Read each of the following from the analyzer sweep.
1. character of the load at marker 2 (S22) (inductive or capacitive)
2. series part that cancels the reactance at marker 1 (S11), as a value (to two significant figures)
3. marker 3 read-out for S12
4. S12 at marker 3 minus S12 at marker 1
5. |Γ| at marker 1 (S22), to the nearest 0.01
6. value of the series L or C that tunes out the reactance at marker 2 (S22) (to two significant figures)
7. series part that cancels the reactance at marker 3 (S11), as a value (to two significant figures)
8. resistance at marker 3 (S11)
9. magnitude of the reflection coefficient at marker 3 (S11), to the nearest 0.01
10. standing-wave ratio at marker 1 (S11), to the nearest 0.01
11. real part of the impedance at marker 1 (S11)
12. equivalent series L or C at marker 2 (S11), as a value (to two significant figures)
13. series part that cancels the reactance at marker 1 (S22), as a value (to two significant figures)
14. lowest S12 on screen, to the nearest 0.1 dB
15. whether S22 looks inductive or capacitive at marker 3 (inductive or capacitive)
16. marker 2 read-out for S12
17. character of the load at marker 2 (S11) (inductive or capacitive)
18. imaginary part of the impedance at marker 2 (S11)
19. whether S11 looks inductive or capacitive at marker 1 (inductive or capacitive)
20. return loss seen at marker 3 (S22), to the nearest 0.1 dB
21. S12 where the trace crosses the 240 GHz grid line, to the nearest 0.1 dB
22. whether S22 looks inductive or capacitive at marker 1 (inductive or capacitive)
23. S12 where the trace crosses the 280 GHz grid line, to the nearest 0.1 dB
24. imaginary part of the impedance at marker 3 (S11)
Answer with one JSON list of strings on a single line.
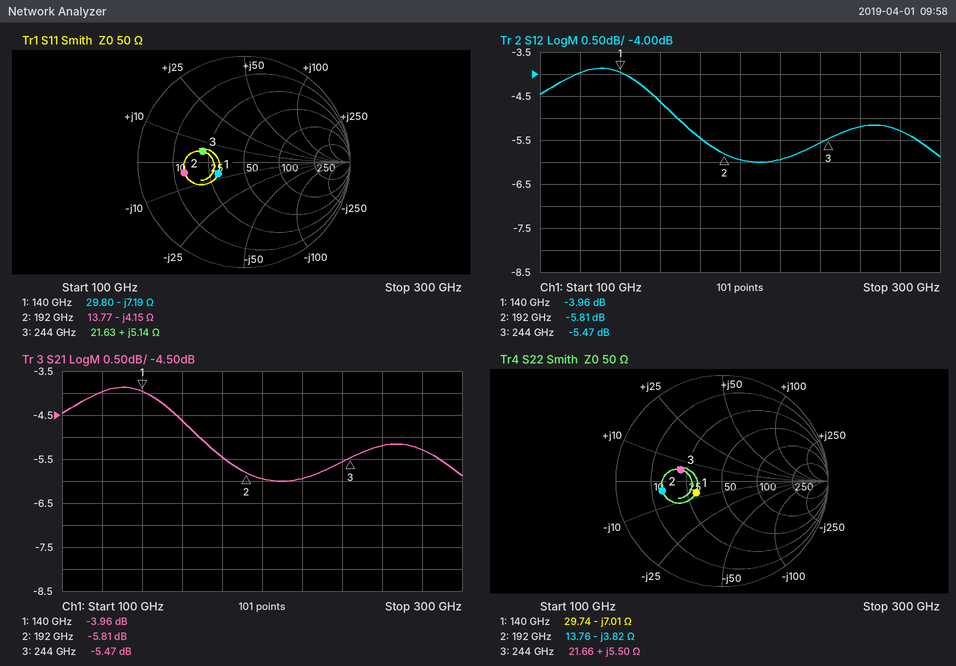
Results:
["capacitive", "8.2 pH", "-5.47 dB", "-1.51 dB", "0.27", "3.2 pH", "130 fF", "21.63 Ω", "0.40", "1.73", "29.80 Ω", "200 fF", "8.0 pH", "-6.0 dB", "inductive", "-5.81 dB", "capacitive", "-4.15 Ω", "capacitive", "7.9 dB", "-5.6 dB", "capacitive", "-5.3 dB", "+5.14 Ω"]
